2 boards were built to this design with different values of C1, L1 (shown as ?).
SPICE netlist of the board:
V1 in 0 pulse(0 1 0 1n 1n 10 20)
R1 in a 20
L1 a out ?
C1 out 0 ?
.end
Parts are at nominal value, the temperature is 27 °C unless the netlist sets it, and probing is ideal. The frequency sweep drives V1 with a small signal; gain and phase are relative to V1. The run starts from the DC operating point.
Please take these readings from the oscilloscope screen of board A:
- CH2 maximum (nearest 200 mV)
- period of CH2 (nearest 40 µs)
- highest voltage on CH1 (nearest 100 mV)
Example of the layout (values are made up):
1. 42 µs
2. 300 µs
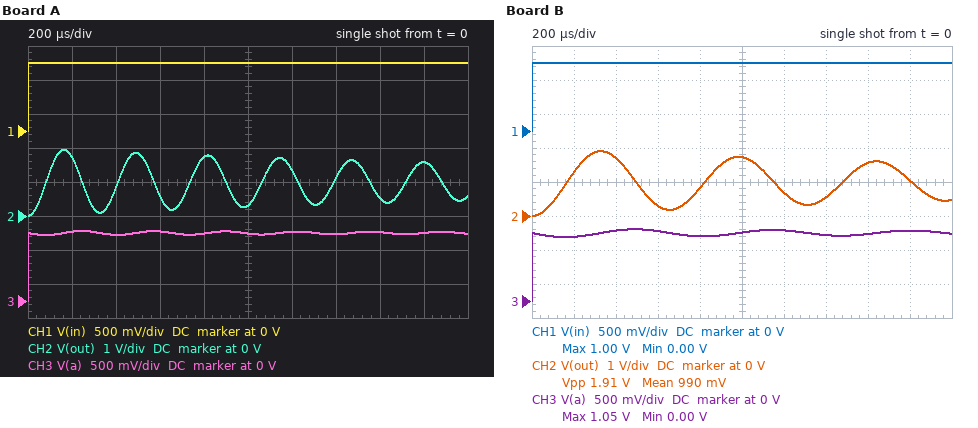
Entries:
1. 2.0 V
2. 320 µs
3. 1.0 V
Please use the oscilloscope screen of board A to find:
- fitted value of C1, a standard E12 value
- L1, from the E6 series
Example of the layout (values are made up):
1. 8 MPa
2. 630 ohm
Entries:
1. 82 nF
2. 33 mH
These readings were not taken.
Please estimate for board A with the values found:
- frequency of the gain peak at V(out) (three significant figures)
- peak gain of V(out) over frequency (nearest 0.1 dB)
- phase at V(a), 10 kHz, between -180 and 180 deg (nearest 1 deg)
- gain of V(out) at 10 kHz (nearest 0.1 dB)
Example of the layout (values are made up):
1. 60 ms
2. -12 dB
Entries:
1. 3.06 kHz
2. 30.0 dB
3. 1 deg
4. -19.7 dB
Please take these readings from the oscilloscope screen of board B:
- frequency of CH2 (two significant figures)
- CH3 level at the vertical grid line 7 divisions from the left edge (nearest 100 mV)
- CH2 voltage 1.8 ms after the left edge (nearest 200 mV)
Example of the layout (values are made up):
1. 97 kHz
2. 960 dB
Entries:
1. 1.5 kHz
2. 1.0 V
3. 1.0 V
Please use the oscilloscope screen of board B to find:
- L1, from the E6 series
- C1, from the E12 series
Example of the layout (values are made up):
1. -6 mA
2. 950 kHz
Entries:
1. 33 mH
2. 330 nF
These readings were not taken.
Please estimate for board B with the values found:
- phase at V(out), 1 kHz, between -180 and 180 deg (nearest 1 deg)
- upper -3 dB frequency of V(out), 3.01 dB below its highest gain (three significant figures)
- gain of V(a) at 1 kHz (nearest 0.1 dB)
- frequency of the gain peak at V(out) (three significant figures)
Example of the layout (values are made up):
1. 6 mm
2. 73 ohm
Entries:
1. -4 deg
2. 1.57 kHz
3. 0 dB
4. 1.52 kHz
